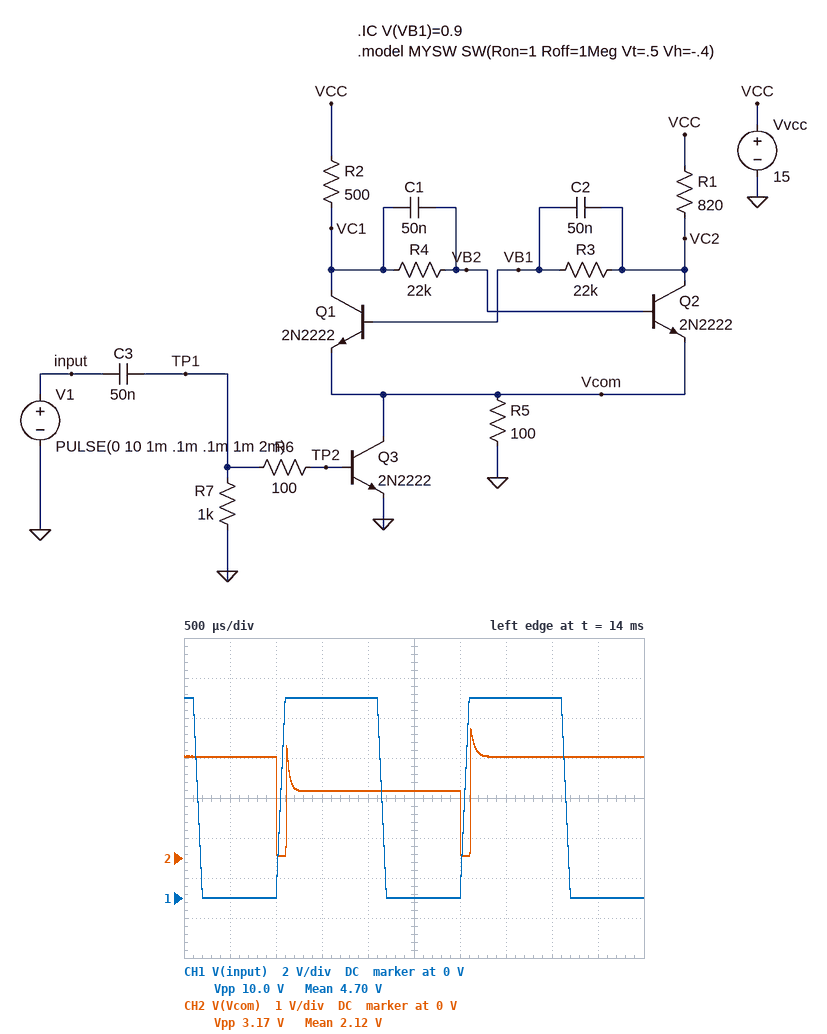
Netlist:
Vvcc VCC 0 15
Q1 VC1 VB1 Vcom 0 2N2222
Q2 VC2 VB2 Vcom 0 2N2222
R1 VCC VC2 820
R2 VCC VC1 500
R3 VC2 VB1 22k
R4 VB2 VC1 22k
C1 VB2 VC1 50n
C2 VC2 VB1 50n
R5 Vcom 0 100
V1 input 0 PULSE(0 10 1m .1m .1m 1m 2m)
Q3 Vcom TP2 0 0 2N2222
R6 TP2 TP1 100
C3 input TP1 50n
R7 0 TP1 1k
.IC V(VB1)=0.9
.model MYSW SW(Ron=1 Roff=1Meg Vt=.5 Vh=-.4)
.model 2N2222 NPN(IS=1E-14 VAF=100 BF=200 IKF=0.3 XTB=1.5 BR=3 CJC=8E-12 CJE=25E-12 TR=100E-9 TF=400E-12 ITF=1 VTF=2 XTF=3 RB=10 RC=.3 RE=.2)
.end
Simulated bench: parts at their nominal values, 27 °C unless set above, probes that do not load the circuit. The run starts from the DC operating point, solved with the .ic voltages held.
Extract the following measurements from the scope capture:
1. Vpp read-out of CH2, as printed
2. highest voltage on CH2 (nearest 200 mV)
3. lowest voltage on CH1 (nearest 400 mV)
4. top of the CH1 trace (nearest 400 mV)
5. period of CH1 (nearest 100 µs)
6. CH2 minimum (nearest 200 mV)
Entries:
3.17 V
3.2 V
0 V
10.0 V
2.0 ms
0 V
